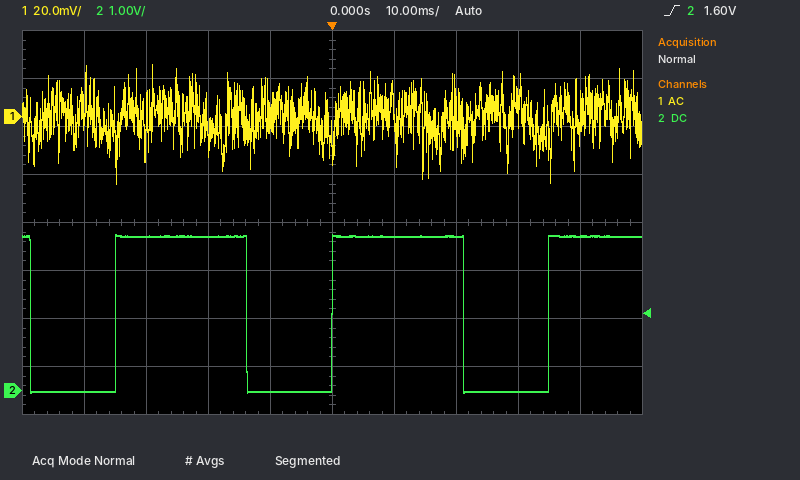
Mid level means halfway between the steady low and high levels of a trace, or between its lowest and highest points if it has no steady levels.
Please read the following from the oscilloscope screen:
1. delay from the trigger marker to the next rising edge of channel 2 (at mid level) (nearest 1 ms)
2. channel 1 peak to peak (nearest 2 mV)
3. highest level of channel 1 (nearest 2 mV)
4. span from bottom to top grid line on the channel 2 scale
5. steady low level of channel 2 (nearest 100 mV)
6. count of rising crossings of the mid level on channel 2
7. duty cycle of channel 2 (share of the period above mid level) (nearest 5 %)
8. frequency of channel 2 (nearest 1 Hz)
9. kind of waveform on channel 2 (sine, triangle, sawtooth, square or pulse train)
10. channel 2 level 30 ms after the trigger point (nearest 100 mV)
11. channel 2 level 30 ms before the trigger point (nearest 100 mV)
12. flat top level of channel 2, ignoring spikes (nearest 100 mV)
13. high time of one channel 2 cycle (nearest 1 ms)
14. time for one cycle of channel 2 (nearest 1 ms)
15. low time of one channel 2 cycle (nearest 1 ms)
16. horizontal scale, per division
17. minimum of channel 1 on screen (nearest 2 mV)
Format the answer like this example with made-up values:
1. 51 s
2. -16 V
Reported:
1. 35 ms
2. 50 mV
3. 22 mV
4. 8 V
5. 0.0 V
6. 3
7. 60 %
8. 29 Hz
9. pulse train
10. 0.0 V
11. 3.2 V
12. 3.2 V
13. 21 ms
14. 35 ms
15. 14 ms
16. 10 ms
17. -28 mV
